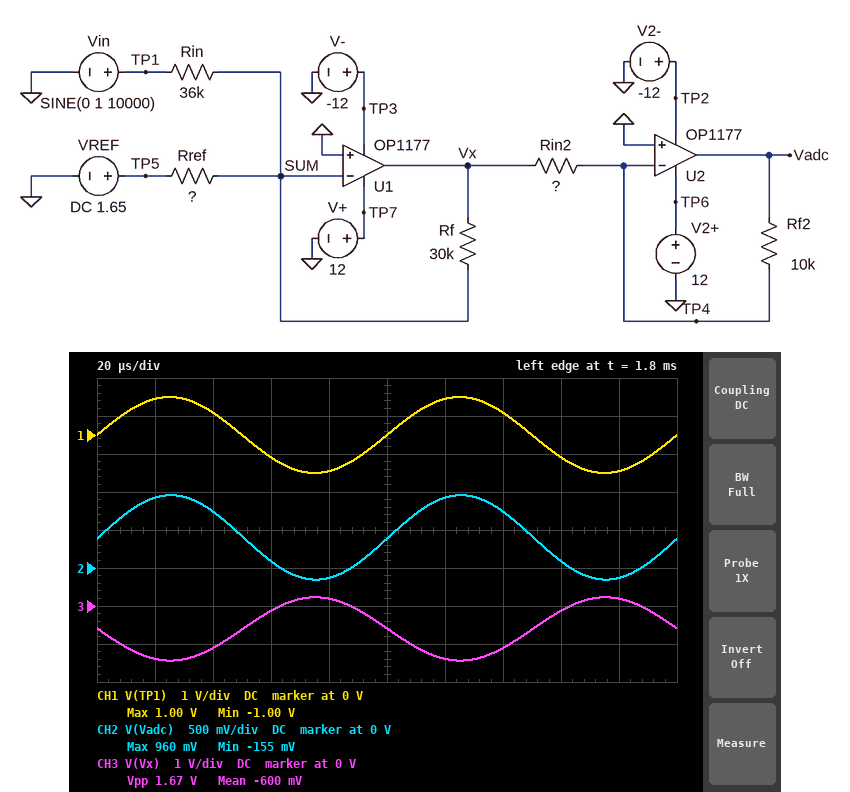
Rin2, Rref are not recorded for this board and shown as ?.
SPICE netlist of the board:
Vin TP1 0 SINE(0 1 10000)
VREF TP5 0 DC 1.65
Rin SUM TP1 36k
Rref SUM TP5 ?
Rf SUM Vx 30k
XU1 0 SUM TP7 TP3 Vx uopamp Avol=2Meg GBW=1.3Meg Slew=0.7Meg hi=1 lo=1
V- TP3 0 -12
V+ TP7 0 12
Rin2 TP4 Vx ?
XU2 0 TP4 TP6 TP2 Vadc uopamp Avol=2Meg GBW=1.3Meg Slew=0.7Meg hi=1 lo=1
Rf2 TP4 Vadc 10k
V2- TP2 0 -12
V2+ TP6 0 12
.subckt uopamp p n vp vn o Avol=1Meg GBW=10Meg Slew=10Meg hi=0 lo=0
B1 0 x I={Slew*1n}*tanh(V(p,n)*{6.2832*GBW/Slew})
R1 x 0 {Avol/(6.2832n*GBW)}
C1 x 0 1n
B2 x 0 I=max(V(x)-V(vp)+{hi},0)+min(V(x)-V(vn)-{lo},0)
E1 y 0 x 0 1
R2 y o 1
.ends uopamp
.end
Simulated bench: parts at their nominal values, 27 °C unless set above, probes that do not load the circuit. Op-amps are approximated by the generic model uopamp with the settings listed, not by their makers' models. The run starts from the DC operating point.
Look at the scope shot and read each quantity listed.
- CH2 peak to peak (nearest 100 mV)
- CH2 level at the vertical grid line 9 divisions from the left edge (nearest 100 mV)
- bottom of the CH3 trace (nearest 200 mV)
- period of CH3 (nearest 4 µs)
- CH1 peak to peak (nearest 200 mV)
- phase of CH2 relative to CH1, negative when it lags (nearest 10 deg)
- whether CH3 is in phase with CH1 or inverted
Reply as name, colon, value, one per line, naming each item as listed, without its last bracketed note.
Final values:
CH2 peak to peak: 1.1 V
CH2 level at the vertical grid line 9 divisions from the left edge: -100 mV
bottom of the CH3 trace: -1.4 V
period of CH3: 100 µs
CH1 peak to peak: 2.0 V
phase of CH2 relative to CH1, negative when it lags: 0 deg
whether CH3 is in phase with CH1 or inverted: inverted
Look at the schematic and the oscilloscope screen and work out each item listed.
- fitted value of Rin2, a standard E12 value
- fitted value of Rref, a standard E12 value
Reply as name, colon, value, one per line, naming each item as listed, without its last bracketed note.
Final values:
fitted value of Rin2, a standard E12 value: 15 kΩ
fitted value of Rref, a standard E12 value: 82 kΩ
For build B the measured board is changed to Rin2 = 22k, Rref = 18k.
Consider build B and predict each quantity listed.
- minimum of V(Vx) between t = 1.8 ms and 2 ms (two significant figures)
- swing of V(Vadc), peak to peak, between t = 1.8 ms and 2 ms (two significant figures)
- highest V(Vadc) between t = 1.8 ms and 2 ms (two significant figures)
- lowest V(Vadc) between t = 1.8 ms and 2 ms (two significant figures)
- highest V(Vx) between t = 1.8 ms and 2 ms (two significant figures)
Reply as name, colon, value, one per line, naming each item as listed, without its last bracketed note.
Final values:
minimum of V(Vx) between t = 1.8 ms and 2 ms: -3.6 V
swing of V(Vadc), peak to peak, between t = 1.8 ms and 2 ms: 760 mV
highest V(Vadc) between t = 1.8 ms and 2 ms: 1.6 V
lowest V(Vadc) between t = 1.8 ms and 2 ms: 870 mV
highest V(Vx) between t = 1.8 ms and 2 ms: -1.9 V
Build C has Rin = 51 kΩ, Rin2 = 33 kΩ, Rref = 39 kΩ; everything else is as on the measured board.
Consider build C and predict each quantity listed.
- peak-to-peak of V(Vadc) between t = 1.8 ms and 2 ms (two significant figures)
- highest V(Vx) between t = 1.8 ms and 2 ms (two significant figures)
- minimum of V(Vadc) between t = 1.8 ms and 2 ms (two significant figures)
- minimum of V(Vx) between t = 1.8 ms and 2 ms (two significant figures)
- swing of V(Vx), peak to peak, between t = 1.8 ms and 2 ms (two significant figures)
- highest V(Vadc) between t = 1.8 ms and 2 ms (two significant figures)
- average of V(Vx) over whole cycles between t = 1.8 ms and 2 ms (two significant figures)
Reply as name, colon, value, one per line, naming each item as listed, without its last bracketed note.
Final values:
peak-to-peak of V(Vadc) between t = 1.8 ms and 2 ms: 360 mV
highest V(Vx) between t = 1.8 ms and 2 ms: -680 mV
minimum of V(Vadc) between t = 1.8 ms and 2 ms: 210 mV
minimum of V(Vx) between t = 1.8 ms and 2 ms: -1.9 V
swing of V(Vx), peak to peak, between t = 1.8 ms and 2 ms: 1.2 V
highest V(Vadc) between t = 1.8 ms and 2 ms: 560 mV
average of V(Vx) over whole cycles between t = 1.8 ms and 2 ms: -1.3 V
